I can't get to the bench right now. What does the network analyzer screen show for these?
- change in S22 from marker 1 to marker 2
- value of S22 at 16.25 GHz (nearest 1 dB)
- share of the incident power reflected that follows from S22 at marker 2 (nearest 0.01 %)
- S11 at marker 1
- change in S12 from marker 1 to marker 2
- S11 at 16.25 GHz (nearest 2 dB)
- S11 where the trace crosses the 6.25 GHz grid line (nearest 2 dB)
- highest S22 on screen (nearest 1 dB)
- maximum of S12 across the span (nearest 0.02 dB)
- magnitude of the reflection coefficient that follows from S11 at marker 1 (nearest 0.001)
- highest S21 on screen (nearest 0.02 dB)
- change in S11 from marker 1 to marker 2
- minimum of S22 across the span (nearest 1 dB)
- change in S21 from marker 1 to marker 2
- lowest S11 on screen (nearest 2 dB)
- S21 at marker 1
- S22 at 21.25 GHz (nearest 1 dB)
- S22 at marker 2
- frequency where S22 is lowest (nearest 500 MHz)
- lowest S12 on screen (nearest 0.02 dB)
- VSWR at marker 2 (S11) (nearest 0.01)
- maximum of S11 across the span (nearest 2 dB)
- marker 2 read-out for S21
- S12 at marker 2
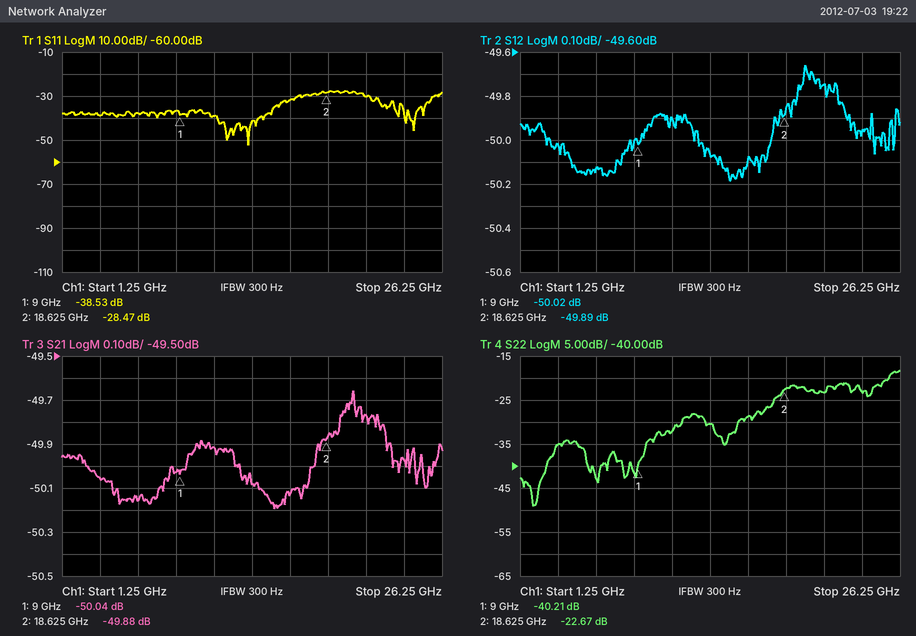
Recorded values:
17.54 dB
-29 dB
0.54 %
-38.53 dB
0.13 dB
-32 dB
-38 dB
-18 dB
-49.66 dB
0.012
-49.66 dB
10.06 dB
-49 dB
0.16 dB
-52 dB
-50.04 dB
-23 dB
-22.67 dB
2.0 GHz
-50.18 dB
1.08
-28 dB
-49.88 dB
-49.89 dB
